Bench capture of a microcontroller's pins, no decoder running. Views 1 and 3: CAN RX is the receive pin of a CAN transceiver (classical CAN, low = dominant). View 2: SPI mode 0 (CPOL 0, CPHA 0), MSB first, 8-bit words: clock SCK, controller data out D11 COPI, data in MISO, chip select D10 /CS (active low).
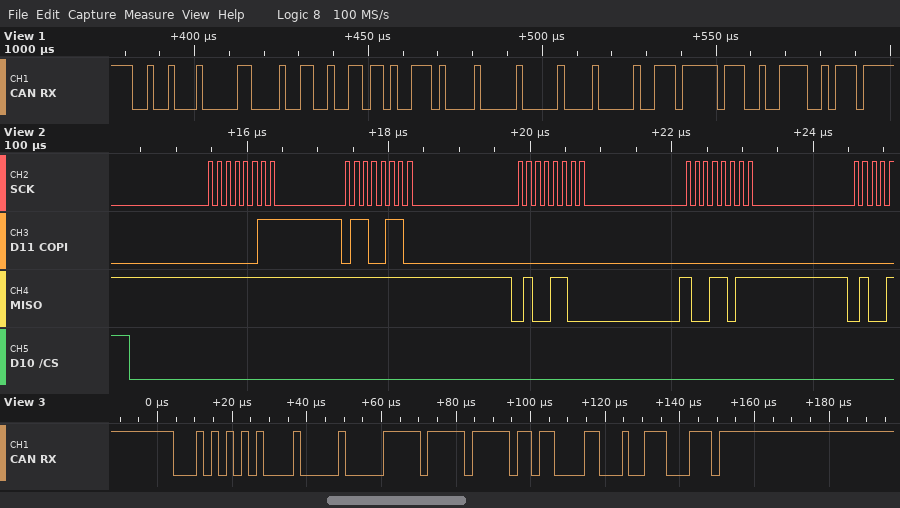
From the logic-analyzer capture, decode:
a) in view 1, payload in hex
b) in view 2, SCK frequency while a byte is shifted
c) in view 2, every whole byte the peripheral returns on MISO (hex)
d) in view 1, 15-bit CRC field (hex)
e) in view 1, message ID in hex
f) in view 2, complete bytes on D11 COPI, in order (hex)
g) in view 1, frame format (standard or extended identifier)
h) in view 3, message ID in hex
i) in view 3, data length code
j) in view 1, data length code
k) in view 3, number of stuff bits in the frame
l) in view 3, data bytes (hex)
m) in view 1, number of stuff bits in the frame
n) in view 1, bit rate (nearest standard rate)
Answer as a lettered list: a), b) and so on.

a) 4C 9B 4E 84 00 08 0E FF
b) 8 MHz
c) FF FF 4C 9B
d) 0x13CB
e) 0x244
f) 03 66 00 00
g) standard
h) 0x155
i) 4
j) 8
k) 5
l) 00 FF FF 61
m) 5
n) 500 kbit/s
